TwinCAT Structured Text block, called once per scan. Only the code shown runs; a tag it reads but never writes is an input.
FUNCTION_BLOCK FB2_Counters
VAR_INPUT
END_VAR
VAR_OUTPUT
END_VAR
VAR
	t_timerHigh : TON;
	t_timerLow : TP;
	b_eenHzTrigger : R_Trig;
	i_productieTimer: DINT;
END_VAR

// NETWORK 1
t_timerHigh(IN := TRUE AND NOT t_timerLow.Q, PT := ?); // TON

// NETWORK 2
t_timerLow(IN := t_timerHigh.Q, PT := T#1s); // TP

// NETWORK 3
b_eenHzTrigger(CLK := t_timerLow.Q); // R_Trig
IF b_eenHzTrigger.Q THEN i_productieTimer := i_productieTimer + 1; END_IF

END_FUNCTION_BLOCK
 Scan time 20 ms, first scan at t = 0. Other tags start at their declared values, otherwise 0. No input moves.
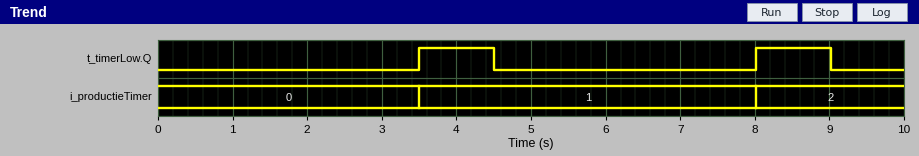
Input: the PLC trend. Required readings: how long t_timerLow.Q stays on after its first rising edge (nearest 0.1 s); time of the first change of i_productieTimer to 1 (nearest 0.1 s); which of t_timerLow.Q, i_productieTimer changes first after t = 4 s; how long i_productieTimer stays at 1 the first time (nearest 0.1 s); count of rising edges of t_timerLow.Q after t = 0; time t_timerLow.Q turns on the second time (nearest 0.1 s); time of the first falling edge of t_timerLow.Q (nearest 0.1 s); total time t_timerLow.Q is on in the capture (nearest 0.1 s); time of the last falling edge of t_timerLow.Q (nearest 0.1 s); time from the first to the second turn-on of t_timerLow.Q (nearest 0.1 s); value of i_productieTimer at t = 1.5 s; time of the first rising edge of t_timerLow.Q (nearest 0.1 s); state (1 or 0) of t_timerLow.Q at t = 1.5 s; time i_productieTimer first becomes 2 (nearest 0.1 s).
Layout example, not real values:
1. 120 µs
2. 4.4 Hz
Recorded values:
1. 1.0 s
2. 3.5 s
3. t_timerLow.Q
4. 4.5 s
5. 2
6. 8.0 s
7. 4.5 s
8. 2.0 s
9. 9.0 s
10. 4.5 s
11. 0
12. 3.5 s
13. 0
14. 8.0 s
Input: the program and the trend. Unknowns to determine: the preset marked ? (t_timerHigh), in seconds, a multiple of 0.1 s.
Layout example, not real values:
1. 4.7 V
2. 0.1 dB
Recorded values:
1. 3.5 s
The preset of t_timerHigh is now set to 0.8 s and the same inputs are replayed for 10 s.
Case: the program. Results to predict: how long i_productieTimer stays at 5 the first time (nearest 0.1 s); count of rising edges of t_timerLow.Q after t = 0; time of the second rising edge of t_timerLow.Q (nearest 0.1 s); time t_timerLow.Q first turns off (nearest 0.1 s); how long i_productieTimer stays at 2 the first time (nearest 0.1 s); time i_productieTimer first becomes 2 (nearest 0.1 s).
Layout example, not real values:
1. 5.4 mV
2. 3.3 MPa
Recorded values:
1. 1.8 s
2. 6
3. 2.6 s
4. 1.8 s
5. 1.8 s
6. 2.6 s
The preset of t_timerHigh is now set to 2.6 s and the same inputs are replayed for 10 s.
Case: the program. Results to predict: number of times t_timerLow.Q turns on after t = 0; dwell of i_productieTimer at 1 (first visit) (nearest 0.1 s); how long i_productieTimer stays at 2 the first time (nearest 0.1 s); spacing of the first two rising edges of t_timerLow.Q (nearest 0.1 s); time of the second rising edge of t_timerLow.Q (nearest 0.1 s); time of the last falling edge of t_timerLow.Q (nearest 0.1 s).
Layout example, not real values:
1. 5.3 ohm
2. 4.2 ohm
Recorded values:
1. 3
2. 3.6 s
3. 3.6 s
4. 3.6 s
5. 6.2 s
6. 7.2 s
